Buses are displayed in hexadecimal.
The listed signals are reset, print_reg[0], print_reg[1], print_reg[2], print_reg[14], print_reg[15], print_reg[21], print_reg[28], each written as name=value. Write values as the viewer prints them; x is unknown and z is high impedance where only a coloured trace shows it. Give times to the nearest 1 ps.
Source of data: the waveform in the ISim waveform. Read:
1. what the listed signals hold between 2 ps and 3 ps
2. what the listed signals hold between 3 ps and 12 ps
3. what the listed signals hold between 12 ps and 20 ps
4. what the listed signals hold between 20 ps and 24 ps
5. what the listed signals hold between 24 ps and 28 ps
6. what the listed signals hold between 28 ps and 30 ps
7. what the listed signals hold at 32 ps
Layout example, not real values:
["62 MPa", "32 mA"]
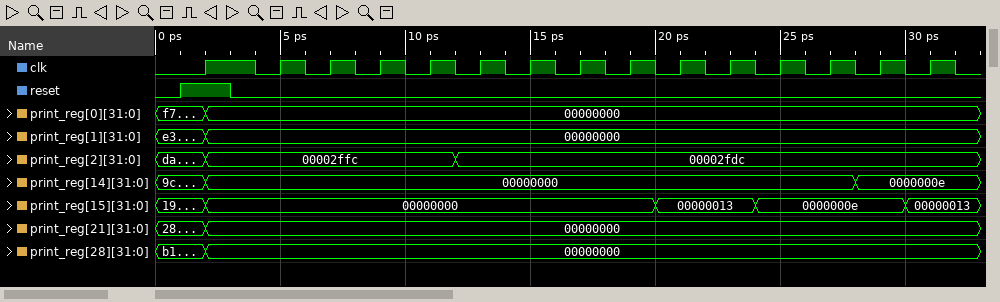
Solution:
["reset=1, print_reg[0]=00000000, print_reg[1]=00000000, print_reg[2]=00002ffc, print_reg[14]=00000000, print_reg[15]=00000000, print_reg[21]=00000000, print_reg[28]=00000000", "reset=0, print_reg[0]=00000000, print_reg[1]=00000000, print_reg[2]=00002ffc, print_reg[14]=00000000, print_reg[15]=00000000, print_reg[21]=00000000, print_reg[28]=00000000", "reset=0, print_reg[0]=00000000, print_reg[1]=00000000, print_reg[2]=00002fdc, print_reg[14]=00000000, print_reg[15]=00000000, print_reg[21]=00000000, print_reg[28]=00000000", "reset=0, print_reg[0]=00000000, print_reg[1]=00000000, print_reg[2]=00002fdc, print_reg[14]=00000000, print_reg[15]=00000013, print_reg[21]=00000000, print_reg[28]=00000000", "reset=0, print_reg[0]=00000000, print_reg[1]=00000000, print_reg[2]=00002fdc, print_reg[14]=00000000, print_reg[15]=0000000e, print_reg[21]=00000000, print_reg[28]=00000000", "reset=0, print_reg[0]=00000000, print_reg[1]=00000000, print_reg[2]=00002fdc, print_reg[14]=0000000e, print_reg[15]=0000000e, print_reg[21]=00000000, print_reg[28]=00000000", "reset=0, print_reg[0]=00000000, print_reg[1]=00000000, print_reg[2]=00002fdc, print_reg[14]=0000000e, print_reg[15]=00000013, print_reg[21]=00000000, print_reg[28]=00000000"]
